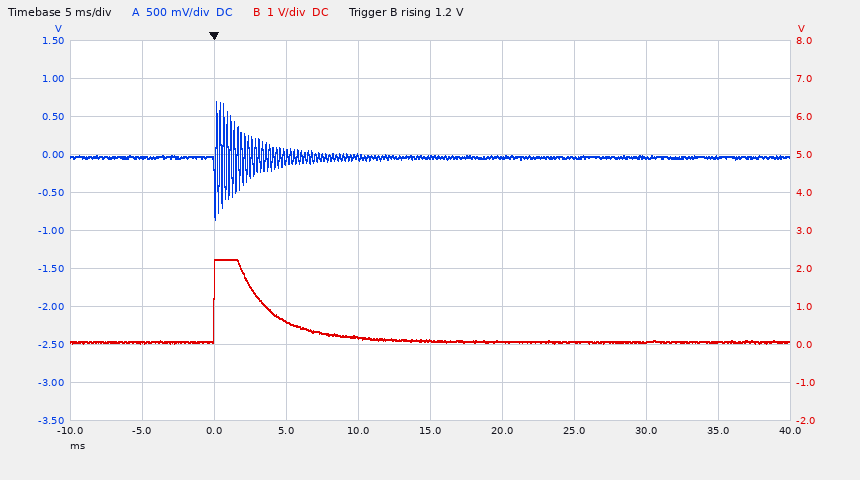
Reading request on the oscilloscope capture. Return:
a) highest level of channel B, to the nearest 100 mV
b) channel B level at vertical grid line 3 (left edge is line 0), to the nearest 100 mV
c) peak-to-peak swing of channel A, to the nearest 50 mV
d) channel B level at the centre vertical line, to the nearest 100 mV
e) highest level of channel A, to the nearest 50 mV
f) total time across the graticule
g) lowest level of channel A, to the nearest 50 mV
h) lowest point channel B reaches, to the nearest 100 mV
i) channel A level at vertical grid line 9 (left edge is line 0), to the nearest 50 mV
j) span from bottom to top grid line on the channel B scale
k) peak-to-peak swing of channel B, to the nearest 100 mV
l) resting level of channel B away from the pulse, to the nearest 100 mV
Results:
2.2 V
600 mV
1.55 V
100 mV
700 mV
50 ms
-850 mV
0.0 V
-50 mV
10 V
2.2 V
100 mV
